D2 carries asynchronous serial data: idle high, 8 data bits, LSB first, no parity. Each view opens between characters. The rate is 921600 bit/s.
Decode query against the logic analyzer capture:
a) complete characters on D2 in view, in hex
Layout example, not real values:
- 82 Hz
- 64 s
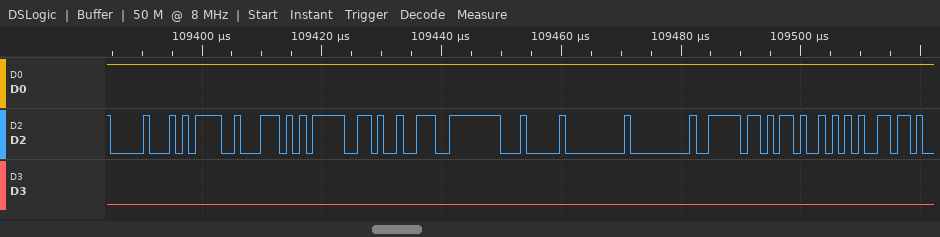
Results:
- 10, 3D, 5C, 9F, C9, FE, 04, 00, 00, BE, 2D, 95
